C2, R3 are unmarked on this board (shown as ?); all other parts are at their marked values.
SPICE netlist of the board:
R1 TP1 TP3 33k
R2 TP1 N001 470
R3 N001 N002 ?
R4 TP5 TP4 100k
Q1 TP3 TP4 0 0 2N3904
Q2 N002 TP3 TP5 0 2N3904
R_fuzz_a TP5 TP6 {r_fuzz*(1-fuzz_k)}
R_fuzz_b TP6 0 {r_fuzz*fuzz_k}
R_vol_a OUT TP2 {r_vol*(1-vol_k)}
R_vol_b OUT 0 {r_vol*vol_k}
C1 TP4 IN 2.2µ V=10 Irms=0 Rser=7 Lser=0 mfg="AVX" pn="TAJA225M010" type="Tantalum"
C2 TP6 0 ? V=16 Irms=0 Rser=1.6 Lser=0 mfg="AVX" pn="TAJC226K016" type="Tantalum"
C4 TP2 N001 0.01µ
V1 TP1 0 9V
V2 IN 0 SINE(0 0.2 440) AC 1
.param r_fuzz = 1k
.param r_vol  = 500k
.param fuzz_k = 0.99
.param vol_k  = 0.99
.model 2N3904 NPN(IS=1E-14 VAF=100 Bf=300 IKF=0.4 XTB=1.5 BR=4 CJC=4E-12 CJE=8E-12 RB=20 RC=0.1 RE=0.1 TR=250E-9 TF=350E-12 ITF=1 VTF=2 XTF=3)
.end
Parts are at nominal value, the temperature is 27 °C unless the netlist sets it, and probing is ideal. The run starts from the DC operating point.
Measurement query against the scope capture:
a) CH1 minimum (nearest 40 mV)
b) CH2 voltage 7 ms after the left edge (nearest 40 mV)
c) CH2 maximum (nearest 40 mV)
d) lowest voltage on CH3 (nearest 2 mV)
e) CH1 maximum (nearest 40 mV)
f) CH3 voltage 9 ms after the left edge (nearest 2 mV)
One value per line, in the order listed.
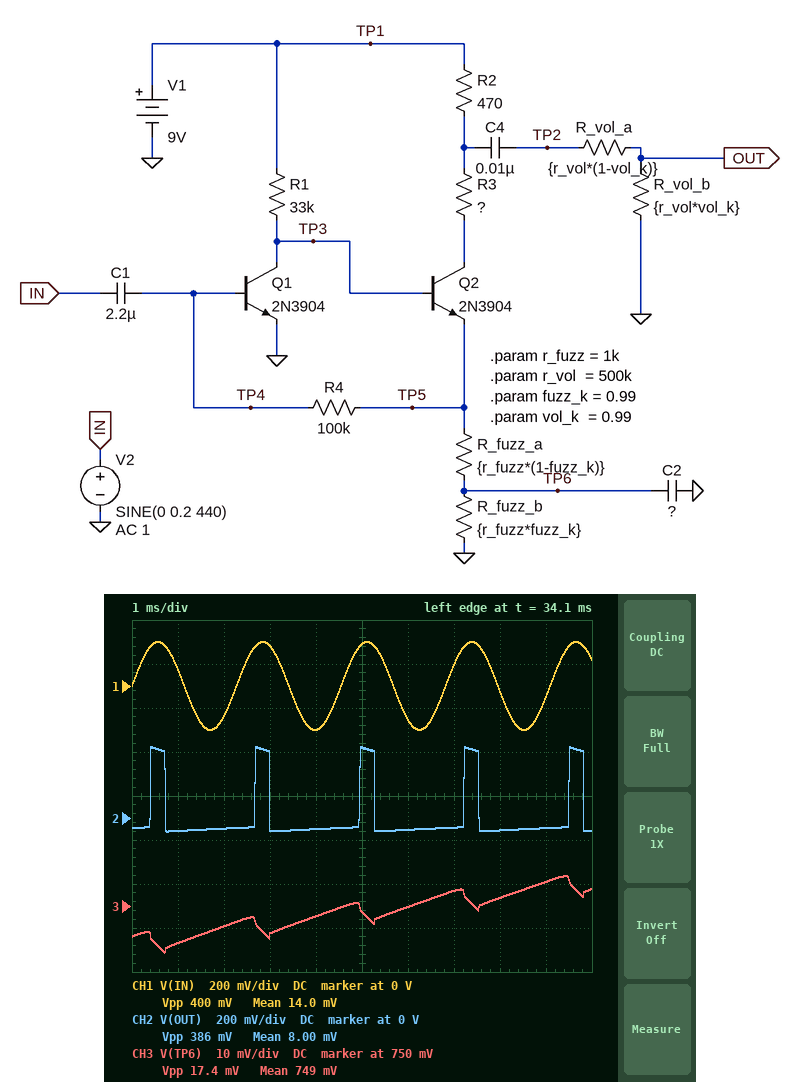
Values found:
-200 mV
-40 mV
320 mV
740 mV
200 mV
756 mV
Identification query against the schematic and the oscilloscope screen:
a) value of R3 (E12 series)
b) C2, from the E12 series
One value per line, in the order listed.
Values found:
10 kΩ
68 µF
